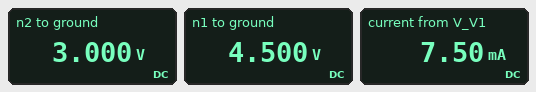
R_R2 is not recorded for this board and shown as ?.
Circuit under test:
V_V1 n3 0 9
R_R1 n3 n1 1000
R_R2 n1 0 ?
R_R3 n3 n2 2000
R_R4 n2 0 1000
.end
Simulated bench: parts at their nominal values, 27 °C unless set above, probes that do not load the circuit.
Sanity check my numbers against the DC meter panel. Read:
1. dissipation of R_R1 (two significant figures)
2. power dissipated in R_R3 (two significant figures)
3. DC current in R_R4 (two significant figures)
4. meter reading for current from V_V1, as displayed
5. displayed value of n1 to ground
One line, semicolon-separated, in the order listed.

20 mW; 18 mW; 3.0 mA; 7.50 mA; 4.500 V
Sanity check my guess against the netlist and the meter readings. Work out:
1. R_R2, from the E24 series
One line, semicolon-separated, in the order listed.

1 kΩ
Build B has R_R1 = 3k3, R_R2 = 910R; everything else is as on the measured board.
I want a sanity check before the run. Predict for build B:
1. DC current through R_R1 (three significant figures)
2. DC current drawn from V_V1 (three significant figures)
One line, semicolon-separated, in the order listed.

2.14 mA; 5.14 mA
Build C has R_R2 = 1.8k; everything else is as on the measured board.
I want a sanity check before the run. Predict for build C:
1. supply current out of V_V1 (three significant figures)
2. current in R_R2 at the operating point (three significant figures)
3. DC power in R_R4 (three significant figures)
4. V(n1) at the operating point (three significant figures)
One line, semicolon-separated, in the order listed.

6.21 mA; 3.21 mA; 9.00 mW; 5.79 V
